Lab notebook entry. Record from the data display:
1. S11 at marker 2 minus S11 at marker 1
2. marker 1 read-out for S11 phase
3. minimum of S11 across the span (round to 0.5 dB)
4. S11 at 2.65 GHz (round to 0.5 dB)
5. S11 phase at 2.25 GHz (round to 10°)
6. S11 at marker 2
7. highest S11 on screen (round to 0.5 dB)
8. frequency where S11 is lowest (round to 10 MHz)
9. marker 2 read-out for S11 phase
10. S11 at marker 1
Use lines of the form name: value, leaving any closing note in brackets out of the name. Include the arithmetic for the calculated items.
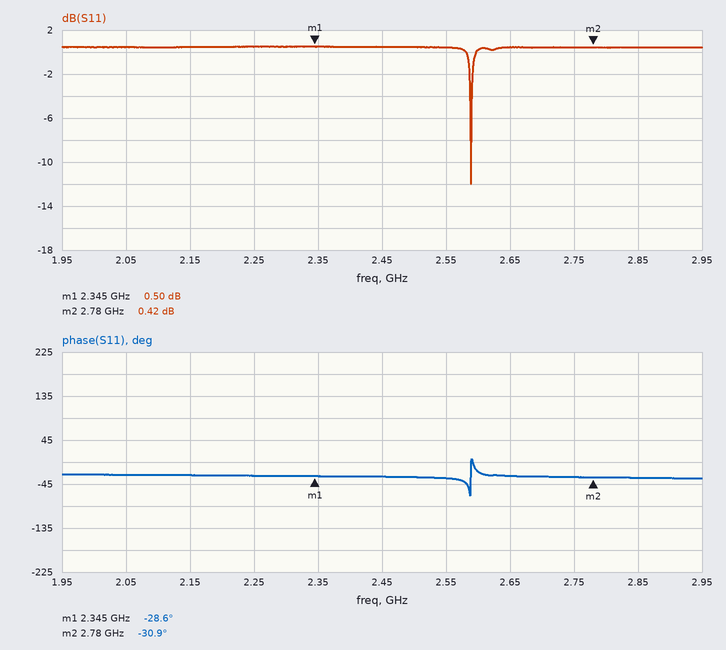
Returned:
S11 at marker 2 minus S11 at marker 1: 0.42 − (0.5) = -0.08 dB
marker 1 read-out for S11 phase: -28.6°
minimum of S11 across the span: -12.0 dB
S11 at 2.65 GHz: 0.5 dB
S11 phase at 2.25 GHz: -30°
S11 at marker 2: 0.42 dB
highest S11 on screen: 0.5 dB
frequency where S11 is lowest: 2.59 GHz
marker 2 read-out for S11 phase: -30.9°
S11 at marker 1: 0.50 dB
